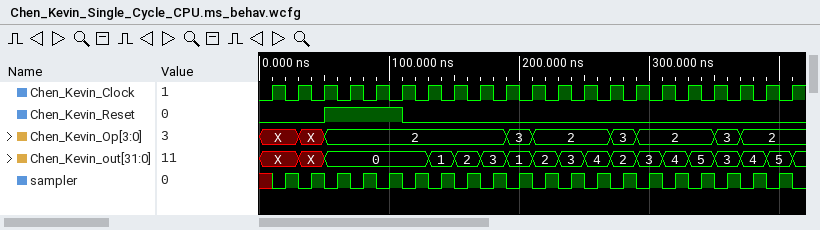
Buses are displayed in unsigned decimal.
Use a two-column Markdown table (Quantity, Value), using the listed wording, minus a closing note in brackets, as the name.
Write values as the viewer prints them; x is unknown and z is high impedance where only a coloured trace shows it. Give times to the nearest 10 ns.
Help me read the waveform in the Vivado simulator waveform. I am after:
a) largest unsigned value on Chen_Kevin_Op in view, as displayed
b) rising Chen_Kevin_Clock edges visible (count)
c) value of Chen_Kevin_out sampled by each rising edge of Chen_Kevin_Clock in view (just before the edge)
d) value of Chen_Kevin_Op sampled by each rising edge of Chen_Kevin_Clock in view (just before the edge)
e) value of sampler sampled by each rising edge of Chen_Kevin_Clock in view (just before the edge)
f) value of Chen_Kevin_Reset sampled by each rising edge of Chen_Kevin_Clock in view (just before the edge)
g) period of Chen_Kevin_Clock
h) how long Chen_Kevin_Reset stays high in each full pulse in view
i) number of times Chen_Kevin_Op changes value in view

| Quantity | Value |
|---|---|
| largest unsigned value on Chen_Kevin_Op in view, as displayed | 3 |
| rising Chen_Kevin_Clock edges visible | 21 |
| value of Chen_Kevin_out sampled by each rising edge of Chen_Kevin_Clock in view | X, X, X, 0, 0, 0, 0, 1, 2, 3, 1, 2, 3, 4, 2, 3, 4, 5, 3, 4, 5 |
| value of Chen_Kevin_Op sampled by each rising edge of Chen_Kevin_Clock in view | X, X, X, 2, 2, 2, 2, 2, 2, 2, 3, 2, 2, 2, 3, 2, 2, 2, 3, 2, 2 |
| value of sampler sampled by each rising edge of Chen_Kevin_Clock in view | x 1 1 1 1 1 1 1 1 1 1 1 1 1 1 1 1 1 1 1 1 |
| value of Chen_Kevin_Reset sampled by each rising edge of Chen_Kevin_Clock in view | 0 0 0 1 1 1 0 0 0 0 0 0 0 0 0 0 0 0 0 0 0 |
| period of Chen_Kevin_Clock | 20 ns |
| how long Chen_Kevin_Reset stays high in each full pulse in view | 60 ns |
| number of times Chen_Kevin_Op changes value in view | 8 |
